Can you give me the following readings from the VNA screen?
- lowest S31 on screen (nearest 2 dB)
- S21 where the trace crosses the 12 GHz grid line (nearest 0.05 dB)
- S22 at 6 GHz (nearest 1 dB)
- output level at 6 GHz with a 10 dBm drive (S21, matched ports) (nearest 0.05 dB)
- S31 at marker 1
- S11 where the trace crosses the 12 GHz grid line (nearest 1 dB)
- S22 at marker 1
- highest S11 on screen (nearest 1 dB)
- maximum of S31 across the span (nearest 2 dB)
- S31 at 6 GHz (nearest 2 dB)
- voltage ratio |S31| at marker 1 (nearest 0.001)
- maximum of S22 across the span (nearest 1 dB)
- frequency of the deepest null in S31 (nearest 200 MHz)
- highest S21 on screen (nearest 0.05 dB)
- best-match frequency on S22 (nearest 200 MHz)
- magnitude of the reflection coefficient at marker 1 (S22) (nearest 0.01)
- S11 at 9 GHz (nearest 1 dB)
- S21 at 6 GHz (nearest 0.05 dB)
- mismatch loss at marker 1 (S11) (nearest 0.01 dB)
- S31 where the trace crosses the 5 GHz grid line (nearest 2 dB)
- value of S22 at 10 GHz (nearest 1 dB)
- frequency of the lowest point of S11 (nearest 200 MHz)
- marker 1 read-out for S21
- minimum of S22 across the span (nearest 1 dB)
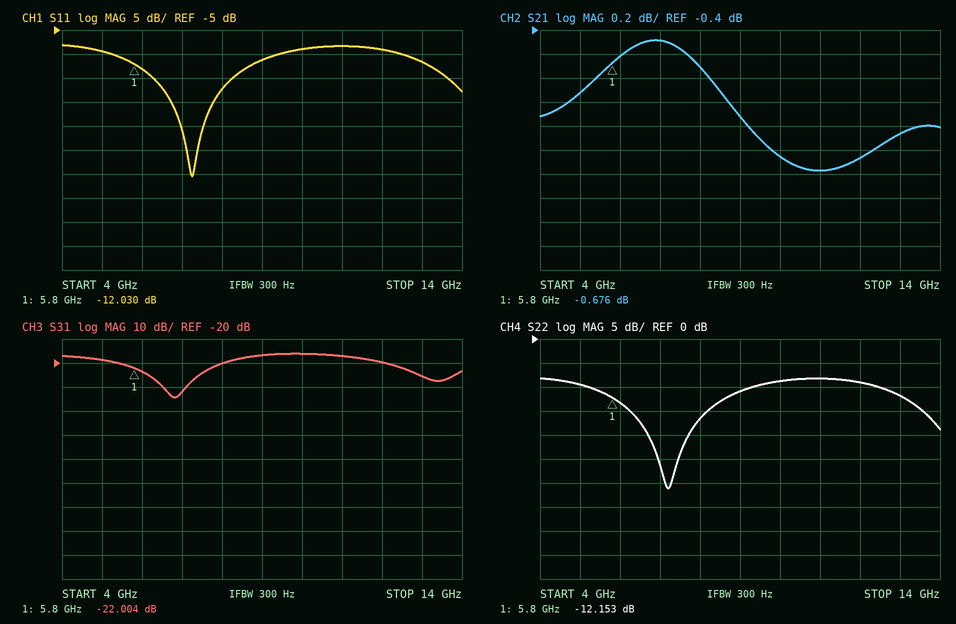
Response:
-34 dB
-1.45 dB
-13 dB
9.40 dBm
-22.004 dB
-9 dB
-12.153 dB
-8 dB
-16 dB
-24 dB
0.079
-8 dB
6.8 GHz
-0.50 dB
7.2 GHz
0.25
-11 dB
-0.60 dB
0.28 dB
-18 dB
-9 dB
7.2 GHz
-0.676 dB
-31 dB
